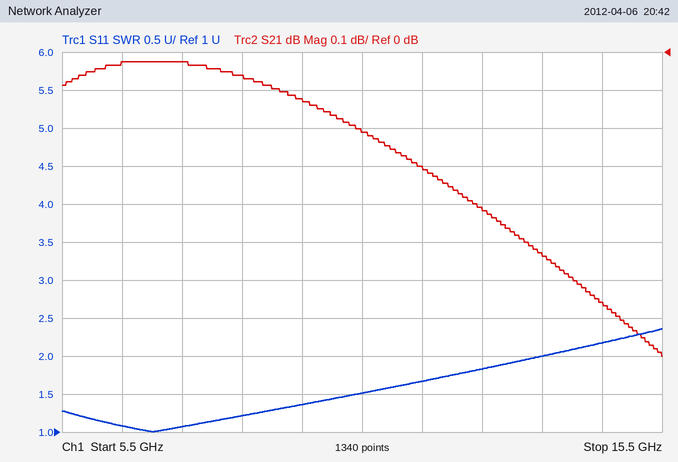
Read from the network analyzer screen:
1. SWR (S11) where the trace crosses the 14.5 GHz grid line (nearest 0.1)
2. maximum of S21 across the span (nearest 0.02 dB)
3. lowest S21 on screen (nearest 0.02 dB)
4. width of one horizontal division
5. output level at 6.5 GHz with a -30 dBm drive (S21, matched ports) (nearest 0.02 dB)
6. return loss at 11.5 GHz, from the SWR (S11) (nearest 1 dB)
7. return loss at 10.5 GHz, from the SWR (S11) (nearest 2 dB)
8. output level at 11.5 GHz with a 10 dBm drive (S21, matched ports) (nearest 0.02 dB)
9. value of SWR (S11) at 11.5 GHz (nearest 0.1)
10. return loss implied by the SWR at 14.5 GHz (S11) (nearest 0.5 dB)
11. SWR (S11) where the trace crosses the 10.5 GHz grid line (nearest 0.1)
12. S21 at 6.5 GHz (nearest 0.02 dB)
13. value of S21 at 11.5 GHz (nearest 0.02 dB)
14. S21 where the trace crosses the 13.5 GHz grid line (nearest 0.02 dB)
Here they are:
2.2
-0.02 dB
-0.80 dB
1 GHz
-30.02 dBm
12 dB
14 dB
9.70 dBm
1.7
8.5 dB
1.5
-0.02 dB
-0.30 dB
-0.54 dB
